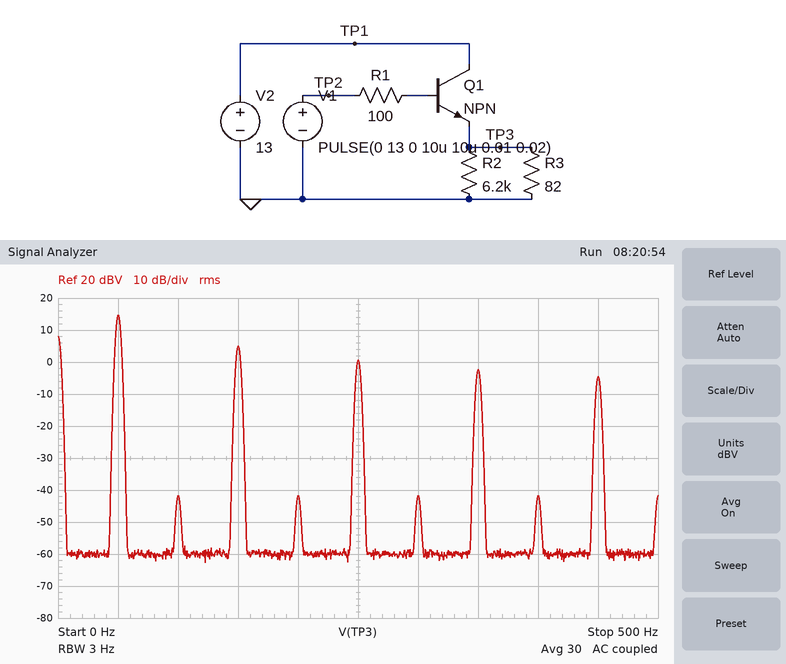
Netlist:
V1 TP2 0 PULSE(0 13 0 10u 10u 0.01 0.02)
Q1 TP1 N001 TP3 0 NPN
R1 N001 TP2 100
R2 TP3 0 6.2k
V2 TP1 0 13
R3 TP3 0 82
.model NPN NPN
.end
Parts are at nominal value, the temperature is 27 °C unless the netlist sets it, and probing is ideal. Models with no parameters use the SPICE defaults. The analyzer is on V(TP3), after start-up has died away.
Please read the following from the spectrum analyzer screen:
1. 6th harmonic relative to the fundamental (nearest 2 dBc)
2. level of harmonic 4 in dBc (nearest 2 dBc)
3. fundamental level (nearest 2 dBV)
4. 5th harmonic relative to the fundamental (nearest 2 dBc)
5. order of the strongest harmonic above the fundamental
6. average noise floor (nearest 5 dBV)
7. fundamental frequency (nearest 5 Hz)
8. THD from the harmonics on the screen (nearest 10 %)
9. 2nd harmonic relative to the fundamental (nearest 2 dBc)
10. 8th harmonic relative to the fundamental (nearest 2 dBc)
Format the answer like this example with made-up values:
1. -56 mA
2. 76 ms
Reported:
1. -56 dBc
2. -56 dBc
3. 14 dBV
4. -14 dBc
5. 3
6. -60 dBV
7. 50 Hz
8. 40 %
9. -56 dBc
10. -56 dBc
